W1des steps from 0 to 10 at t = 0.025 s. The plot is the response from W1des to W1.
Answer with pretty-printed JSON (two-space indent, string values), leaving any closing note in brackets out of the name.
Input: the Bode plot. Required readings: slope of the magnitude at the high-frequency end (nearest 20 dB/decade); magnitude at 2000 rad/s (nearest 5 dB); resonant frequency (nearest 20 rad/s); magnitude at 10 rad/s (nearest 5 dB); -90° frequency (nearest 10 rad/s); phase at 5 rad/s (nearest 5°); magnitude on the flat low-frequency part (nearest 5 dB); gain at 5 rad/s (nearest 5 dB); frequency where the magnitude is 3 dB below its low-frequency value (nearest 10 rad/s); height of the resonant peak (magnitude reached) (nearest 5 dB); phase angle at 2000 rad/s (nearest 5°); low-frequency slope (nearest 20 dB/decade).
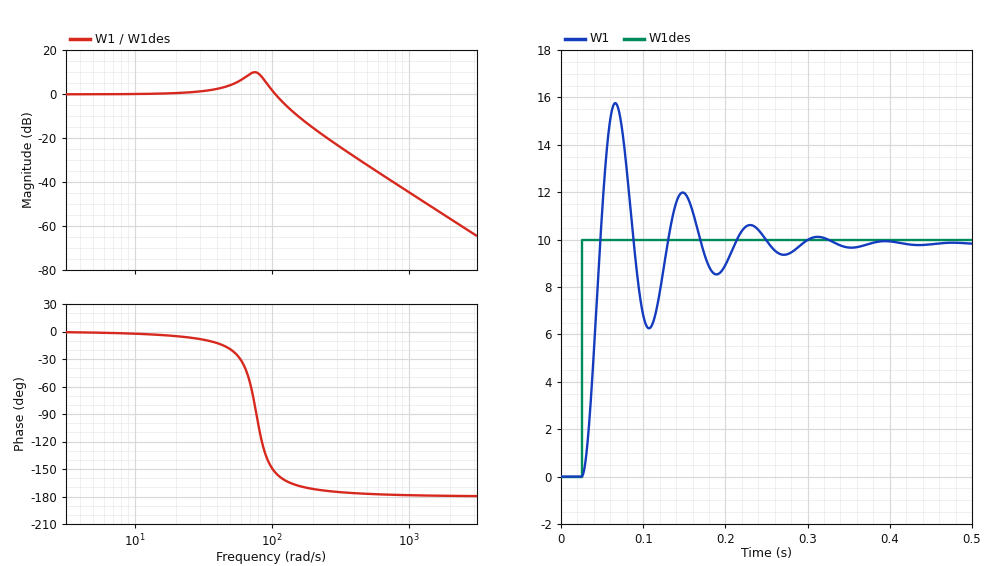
{
  "slope of the magnitude at the high-frequency end": "-40 dB/decade",
  "magnitude at 2000 rad/s": "-55 dB",
  "resonant frequency": "80 rad/s",
  "magnitude at 10 rad/s": "0 dB",
  "-90° frequency": "80 rad/s",
  "phase at 5 rad/s": "0°",
  "magnitude on the flat low-frequency part": "0 dB",
  "gain at 5 rad/s": "0 dB",
  "frequency where the magnitude is 3 dB below its low-frequency value": "120 rad/s",
  "height of the resonant peak (magnitude reached)": "10 dB",
  "phase angle at 2000 rad/s": "-180°",
  "low-frequency slope": "0 dB/decade"
}
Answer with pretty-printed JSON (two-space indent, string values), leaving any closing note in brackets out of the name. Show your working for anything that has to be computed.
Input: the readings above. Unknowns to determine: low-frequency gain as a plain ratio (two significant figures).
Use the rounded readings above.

{
  "low-frequency gain as a plain ratio": "10^(0 / 20) = 1.0"
}
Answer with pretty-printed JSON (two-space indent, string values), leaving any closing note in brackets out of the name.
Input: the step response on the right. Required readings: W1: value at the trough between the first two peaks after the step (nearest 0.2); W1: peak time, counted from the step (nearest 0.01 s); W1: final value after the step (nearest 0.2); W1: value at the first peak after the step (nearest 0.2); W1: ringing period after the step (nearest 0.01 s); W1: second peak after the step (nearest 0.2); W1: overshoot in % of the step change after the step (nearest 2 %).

{
  "W1: value at the trough between the first two peaks after the step": "6.2",
  "W1: peak time, counted from the step": "0.04 s",
  "W1: final value after the step": "9.8",
  "W1: value at the first peak after the step": "15.8",
  "W1: ringing period after the step": "0.08 s",
  "W1: second peak after the step": "12.0",
  "W1: overshoot in % of the step change after the step": "60 %"
}
